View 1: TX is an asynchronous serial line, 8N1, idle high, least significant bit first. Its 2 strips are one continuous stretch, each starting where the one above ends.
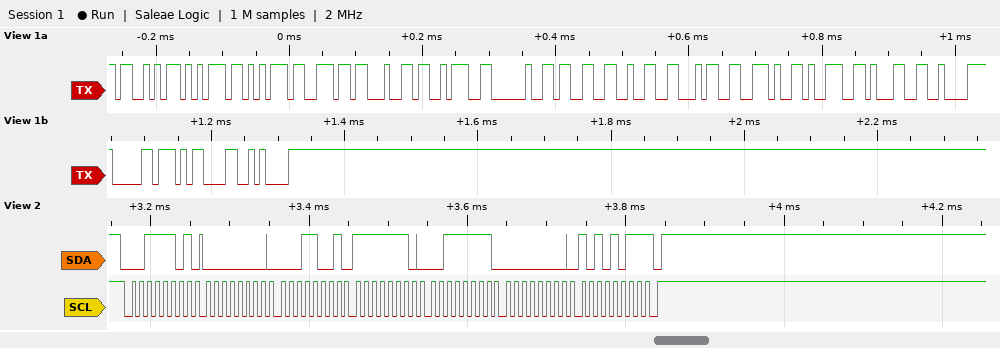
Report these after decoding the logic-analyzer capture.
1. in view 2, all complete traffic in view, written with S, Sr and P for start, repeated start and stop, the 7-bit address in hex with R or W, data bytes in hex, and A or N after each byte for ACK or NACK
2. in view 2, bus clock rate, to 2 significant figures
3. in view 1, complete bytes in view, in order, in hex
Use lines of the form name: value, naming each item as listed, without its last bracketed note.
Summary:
in view 2, all complete traffic in view, written with S, Sr and P for start, repeated start and stop, the 7-bit address in hex with R or W, data bytes in hex, and A or N after each byte for ACK or NACK: S 1ER A 00 A 19 A FE A 3F A 00 A AB N P
in view 2, bus clock rate, to 2 significant figures: 100 kHz
in view 1, complete bytes in view, in order, in hex: 53 75 75 6E 64 3A 20 33 32 34 2E 39 31 C2 B0 0D 0A
